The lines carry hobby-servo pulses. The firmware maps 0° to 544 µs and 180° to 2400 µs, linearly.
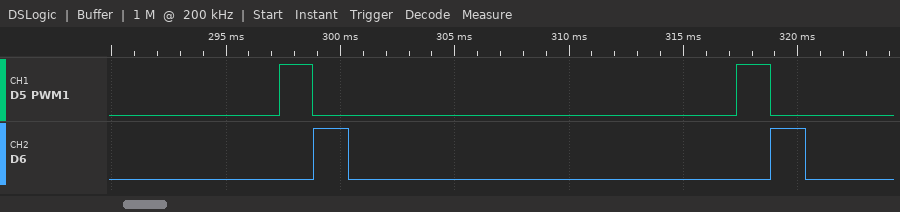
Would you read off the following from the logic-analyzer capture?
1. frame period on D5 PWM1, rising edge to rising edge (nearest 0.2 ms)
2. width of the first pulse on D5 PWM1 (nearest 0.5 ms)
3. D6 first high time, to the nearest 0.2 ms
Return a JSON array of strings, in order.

["20.0 ms", "1.5 ms", "1.6 ms"]
